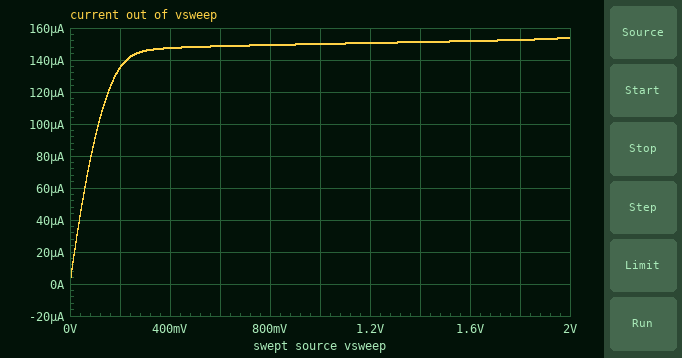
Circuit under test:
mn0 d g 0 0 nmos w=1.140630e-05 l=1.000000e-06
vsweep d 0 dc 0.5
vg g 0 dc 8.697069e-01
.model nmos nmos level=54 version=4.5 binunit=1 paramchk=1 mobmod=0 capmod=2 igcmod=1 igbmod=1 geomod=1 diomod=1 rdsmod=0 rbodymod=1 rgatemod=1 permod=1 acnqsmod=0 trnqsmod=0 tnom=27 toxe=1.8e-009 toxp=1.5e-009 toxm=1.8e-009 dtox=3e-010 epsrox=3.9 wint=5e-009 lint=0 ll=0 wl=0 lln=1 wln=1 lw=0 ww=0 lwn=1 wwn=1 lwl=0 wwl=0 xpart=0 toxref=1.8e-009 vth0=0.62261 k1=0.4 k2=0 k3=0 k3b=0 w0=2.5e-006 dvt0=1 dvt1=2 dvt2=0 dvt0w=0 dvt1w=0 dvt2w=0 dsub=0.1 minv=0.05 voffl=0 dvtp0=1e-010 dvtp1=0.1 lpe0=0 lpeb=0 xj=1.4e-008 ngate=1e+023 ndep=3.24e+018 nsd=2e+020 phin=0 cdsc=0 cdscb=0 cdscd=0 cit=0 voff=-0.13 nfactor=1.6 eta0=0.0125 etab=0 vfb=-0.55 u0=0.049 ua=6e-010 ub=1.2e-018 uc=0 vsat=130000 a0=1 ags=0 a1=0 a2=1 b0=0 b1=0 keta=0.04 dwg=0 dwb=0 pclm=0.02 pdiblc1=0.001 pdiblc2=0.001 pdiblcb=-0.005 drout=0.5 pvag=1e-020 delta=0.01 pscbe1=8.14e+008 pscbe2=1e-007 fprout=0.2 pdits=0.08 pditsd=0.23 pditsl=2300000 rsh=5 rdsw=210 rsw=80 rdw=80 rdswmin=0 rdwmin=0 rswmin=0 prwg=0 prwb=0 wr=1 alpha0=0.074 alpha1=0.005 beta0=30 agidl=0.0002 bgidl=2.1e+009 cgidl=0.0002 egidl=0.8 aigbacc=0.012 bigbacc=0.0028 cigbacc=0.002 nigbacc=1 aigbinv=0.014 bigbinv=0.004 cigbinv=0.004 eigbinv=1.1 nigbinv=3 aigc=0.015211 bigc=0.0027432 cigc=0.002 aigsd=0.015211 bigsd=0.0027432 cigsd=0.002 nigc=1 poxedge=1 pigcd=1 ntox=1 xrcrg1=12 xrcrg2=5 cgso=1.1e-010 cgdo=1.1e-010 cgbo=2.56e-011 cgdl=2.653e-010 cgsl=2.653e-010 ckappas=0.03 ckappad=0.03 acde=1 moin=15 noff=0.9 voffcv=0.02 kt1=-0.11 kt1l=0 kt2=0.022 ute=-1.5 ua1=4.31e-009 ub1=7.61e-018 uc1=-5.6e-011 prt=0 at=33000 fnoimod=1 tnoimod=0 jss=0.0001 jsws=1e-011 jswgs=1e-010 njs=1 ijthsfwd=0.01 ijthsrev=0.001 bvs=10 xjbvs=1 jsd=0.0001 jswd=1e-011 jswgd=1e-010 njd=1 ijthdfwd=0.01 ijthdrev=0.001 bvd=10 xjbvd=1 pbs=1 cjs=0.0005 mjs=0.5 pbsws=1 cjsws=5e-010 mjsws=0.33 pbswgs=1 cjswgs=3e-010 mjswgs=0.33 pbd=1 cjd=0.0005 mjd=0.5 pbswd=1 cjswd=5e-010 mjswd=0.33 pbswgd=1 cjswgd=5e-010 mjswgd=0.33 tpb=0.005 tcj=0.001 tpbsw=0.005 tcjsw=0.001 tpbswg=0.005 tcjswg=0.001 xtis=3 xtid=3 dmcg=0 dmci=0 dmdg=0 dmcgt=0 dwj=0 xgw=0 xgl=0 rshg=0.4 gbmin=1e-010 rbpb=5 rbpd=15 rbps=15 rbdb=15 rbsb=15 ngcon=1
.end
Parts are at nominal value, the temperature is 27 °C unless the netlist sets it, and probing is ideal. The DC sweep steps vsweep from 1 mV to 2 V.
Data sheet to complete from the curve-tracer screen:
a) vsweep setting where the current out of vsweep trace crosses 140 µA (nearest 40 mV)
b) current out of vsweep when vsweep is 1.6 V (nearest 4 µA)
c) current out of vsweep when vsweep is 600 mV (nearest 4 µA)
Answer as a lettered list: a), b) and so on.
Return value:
a) 240 mV
b) 152 µA
c) 148 µA
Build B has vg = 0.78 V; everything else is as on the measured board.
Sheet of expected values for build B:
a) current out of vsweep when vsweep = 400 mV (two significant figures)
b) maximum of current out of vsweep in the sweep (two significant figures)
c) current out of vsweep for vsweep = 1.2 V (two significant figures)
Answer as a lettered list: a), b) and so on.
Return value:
a) 72 µA
b) 75 µA
c) 73 µA
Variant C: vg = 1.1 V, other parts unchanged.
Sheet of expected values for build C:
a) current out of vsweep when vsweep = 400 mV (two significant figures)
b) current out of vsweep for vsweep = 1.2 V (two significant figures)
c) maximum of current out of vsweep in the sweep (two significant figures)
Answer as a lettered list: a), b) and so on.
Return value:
a) 420 µA
b) 440 µA
c) 450 µA
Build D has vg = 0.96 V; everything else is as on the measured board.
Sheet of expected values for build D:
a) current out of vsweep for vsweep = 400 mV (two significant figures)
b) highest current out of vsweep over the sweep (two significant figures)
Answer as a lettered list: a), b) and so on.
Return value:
a) 250 µA
b) 260 µA
